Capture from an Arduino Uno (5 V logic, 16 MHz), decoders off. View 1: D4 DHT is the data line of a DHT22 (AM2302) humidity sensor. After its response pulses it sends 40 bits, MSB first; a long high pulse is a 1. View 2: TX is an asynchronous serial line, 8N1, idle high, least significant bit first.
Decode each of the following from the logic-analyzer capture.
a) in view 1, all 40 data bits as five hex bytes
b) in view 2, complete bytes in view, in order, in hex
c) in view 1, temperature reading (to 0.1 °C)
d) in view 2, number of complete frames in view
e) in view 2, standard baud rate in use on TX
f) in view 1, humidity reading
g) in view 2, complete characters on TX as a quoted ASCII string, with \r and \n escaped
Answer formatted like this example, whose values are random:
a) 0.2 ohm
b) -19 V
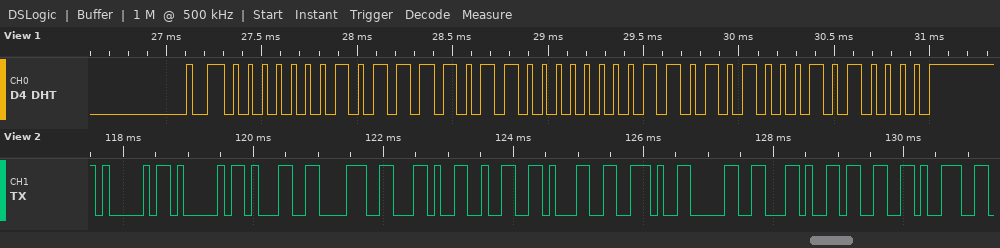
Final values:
a) 01 7B 00 D4 50
b) 0x41 0x41 0x31 0x38 0x2C 0x32 0x31 0x2E 0x30 0x2C 0x33 0x39
c) 21.2 °C
d) 12
e) 9600 baud
f) 37.9 %
g) "AA18,21.0,39"
